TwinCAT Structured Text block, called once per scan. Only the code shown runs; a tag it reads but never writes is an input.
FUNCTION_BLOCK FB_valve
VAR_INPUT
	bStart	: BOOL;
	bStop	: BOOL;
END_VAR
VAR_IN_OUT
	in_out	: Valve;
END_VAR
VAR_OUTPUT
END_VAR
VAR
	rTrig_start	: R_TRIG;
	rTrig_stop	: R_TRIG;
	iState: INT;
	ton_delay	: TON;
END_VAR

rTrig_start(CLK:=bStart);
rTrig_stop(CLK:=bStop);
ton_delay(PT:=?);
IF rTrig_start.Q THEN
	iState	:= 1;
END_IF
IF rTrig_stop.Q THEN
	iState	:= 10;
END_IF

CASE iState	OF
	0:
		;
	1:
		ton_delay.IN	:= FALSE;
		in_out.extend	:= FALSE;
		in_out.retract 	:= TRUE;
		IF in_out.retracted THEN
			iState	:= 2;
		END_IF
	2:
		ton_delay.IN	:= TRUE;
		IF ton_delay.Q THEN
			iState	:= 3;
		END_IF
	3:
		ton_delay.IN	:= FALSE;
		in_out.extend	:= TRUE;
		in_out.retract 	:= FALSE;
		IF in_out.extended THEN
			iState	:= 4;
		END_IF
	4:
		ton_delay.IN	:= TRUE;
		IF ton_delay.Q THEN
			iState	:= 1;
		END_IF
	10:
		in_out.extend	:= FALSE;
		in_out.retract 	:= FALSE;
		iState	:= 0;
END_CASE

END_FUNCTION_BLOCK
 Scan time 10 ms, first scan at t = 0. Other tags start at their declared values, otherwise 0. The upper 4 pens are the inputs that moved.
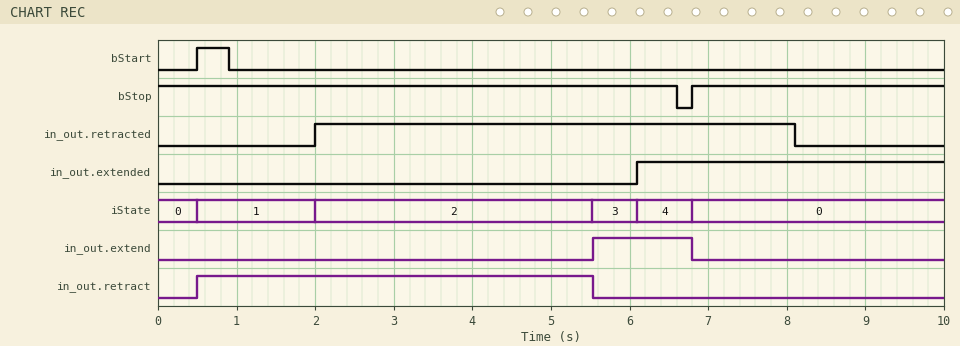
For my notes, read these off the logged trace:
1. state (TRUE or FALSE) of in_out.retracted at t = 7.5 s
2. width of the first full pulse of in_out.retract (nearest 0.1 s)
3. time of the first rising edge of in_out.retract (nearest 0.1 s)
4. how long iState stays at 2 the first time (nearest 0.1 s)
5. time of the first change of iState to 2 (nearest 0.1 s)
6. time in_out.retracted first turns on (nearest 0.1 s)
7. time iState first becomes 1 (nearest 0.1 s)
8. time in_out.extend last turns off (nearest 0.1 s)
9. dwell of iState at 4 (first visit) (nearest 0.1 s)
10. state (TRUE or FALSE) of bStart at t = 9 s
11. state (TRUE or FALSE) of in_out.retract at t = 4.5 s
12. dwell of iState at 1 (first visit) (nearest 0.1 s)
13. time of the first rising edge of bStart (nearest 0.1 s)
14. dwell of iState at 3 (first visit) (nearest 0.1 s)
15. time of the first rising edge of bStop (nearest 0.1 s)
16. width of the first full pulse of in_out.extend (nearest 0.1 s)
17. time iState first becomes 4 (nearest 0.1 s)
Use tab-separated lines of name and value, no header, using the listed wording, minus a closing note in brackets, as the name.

state (TRUE or FALSE) of in_out.retracted at t = 7.5 s	TRUE
width of the first full pulse of in_out.retract	5.0 s
time of the first rising edge of in_out.retract	0.5 s
how long iState stays at 2 the first time	3.5 s
time of the first change of iState to 2	2.0 s
time in_out.retracted first turns on	2.0 s
time iState first becomes 1	0.5 s
time in_out.extend last turns off	6.8 s
dwell of iState at 4 (first visit)	0.7 s
state (TRUE or FALSE) of bStart at t = 9 s	FALSE
state (TRUE or FALSE) of in_out.retract at t = 4.5 s	TRUE
dwell of iState at 1 (first visit)	1.5 s
time of the first rising edge of bStart	0.5 s
dwell of iState at 3 (first visit)	0.6 s
time of the first rising edge of bStop	6.8 s
width of the first full pulse of in_out.extend	1.3 s
time iState first becomes 4	6.1 s
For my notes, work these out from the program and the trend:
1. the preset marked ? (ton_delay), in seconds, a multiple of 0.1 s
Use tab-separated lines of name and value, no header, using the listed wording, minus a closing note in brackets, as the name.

the preset marked ? (ton_delay), in seconds, a multiple of 0.1 s	3.5 s
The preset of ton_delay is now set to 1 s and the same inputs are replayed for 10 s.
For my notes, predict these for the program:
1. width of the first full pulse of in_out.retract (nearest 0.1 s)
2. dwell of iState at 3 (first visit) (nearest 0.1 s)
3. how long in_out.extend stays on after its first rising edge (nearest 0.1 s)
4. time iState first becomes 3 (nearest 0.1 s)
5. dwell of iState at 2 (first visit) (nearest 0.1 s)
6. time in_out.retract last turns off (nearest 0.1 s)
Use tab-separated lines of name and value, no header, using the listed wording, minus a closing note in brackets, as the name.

width of the first full pulse of in_out.retract	2.5 s
dwell of iState at 3 (first visit)	3.1 s
how long in_out.extend stays on after its first rising edge	3.8 s
time iState first becomes 3	3.0 s
dwell of iState at 2 (first visit)	1.0 s
time in_out.retract last turns off	3.0 s
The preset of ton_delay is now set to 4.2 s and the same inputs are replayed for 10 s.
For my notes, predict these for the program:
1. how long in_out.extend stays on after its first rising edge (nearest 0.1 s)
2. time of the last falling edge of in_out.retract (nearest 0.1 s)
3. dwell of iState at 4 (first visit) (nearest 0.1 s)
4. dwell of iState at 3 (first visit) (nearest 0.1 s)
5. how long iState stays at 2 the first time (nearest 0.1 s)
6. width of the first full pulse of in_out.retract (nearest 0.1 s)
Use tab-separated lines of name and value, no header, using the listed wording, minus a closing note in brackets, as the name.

how long in_out.extend stays on after its first rising edge	0.6 s
time of the last falling edge of in_out.retract	6.2 s
dwell of iState at 4 (first visit)	0.6 s
dwell of iState at 3 (first visit)	0.0 s
how long iState stays at 2 the first time	4.2 s
width of the first full pulse of in_out.retract	5.7 s
